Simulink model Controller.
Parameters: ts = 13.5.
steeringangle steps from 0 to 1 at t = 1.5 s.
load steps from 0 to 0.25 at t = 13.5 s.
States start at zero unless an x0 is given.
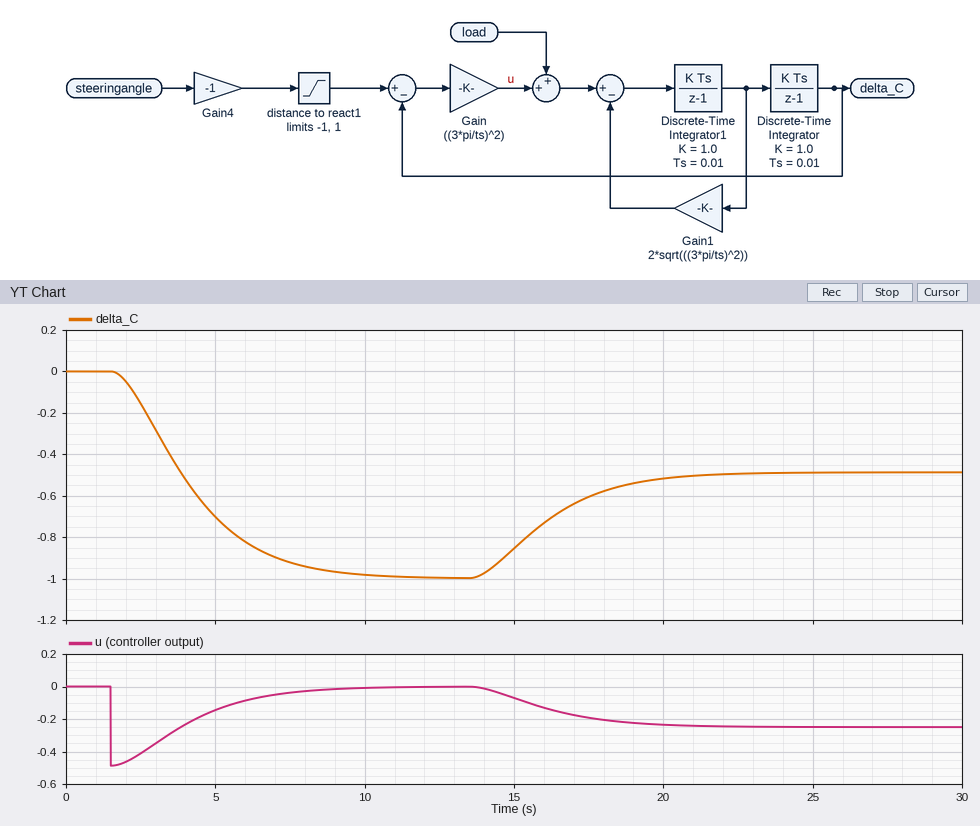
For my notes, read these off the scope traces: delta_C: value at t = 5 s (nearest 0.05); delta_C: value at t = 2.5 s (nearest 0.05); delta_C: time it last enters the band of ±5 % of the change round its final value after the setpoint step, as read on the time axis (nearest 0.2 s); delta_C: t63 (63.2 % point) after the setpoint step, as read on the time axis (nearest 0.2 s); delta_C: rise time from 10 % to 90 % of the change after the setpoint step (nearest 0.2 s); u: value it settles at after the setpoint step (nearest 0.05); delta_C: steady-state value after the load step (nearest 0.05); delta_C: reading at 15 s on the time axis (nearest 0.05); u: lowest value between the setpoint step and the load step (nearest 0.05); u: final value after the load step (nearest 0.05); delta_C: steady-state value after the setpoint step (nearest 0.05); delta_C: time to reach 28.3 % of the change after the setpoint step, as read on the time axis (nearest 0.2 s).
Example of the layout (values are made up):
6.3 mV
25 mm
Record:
-0.70
-0.15
8.2 s
4.6 s
4.8 s
0.00
-0.50
-0.85
-0.50
-0.25
-1.00
3.0 s
